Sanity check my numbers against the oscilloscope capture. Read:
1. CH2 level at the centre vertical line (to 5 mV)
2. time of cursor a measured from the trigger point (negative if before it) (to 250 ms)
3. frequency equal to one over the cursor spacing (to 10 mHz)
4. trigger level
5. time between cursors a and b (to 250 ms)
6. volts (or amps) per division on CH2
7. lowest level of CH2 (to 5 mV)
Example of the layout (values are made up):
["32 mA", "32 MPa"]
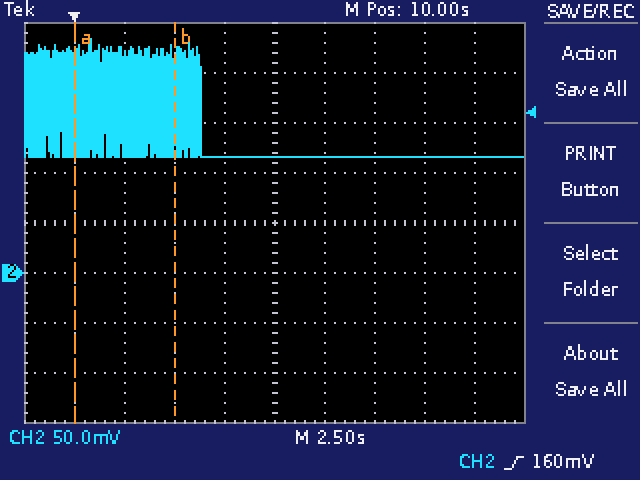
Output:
["115 mV", "0.00 s", "200 mHz", "160 mV", "5.00 s", "50 mV", "115 mV"]
